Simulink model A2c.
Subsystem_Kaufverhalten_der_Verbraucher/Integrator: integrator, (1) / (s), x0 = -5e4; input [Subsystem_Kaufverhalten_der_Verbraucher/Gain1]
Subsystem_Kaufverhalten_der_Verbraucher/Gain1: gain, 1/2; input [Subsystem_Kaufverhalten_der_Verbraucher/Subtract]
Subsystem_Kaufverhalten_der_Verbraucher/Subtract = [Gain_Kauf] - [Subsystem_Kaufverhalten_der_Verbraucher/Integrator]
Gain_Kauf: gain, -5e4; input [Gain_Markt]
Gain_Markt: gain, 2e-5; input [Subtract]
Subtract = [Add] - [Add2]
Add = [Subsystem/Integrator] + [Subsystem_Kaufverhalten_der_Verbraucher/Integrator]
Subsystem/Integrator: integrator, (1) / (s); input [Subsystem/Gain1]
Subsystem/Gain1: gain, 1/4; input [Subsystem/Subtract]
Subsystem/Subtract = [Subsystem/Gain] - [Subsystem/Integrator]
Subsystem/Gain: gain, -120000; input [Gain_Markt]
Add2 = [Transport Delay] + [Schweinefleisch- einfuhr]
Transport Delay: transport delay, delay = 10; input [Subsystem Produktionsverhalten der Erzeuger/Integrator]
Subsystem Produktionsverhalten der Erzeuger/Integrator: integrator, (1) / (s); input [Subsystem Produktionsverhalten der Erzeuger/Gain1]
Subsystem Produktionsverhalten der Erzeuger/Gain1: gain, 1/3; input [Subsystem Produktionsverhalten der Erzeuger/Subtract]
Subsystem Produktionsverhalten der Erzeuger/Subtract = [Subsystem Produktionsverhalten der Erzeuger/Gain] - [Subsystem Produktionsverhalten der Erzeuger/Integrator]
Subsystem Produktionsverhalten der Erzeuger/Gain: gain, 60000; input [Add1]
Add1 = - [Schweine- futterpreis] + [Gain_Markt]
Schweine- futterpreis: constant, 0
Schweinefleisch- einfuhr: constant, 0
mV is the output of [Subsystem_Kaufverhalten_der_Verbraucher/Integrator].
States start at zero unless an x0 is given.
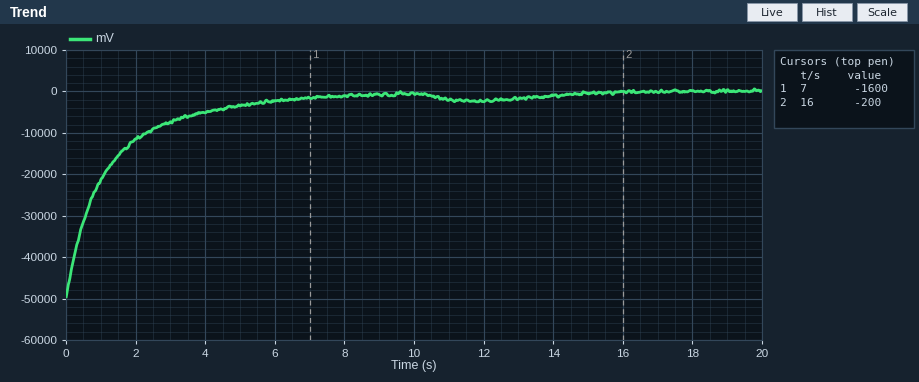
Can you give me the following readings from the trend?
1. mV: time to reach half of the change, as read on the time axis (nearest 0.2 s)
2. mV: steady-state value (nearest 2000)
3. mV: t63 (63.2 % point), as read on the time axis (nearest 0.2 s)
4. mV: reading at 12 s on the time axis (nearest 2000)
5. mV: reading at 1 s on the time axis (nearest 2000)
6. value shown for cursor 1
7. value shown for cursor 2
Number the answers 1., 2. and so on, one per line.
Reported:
1. 0.8 s
2. 0
3. 1.2 s
4. -2000
5. -22000
6. -1600
7. -200
